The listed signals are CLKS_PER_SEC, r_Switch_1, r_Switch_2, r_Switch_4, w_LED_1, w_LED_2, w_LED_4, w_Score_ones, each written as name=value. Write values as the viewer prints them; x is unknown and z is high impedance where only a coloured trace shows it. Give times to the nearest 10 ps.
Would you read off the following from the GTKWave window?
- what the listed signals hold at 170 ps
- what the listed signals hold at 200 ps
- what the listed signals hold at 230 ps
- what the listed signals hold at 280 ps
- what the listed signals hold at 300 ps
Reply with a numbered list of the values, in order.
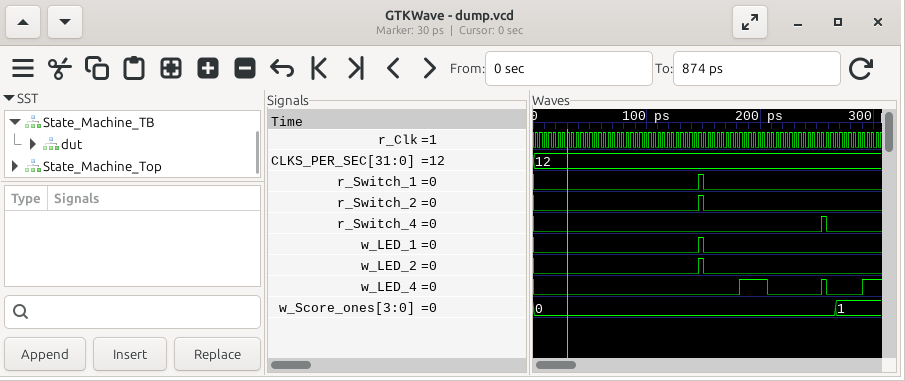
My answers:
1. CLKS_PER_SEC=12, r_Switch_1=0, r_Switch_2=0, r_Switch_4=0, w_LED_1=0, w_LED_2=0, w_LED_4=0, w_Score_ones=0
2. CLKS_PER_SEC=12, r_Switch_1=0, r_Switch_2=0, r_Switch_4=0, w_LED_1=0, w_LED_2=0, w_LED_4=1, w_Score_ones=0
3. CLKS_PER_SEC=12, r_Switch_1=0, r_Switch_2=0, r_Switch_4=0, w_LED_1=0, w_LED_2=0, w_LED_4=0, w_Score_ones=0
4. CLKS_PER_SEC=12, r_Switch_1=0, r_Switch_2=0, r_Switch_4=0, w_LED_1=0, w_LED_2=0, w_LED_4=0, w_Score_ones=1
5. CLKS_PER_SEC=12, r_Switch_1=0, r_Switch_2=0, r_Switch_4=0, w_LED_1=0, w_LED_2=0, w_LED_4=1, w_Score_ones=1
